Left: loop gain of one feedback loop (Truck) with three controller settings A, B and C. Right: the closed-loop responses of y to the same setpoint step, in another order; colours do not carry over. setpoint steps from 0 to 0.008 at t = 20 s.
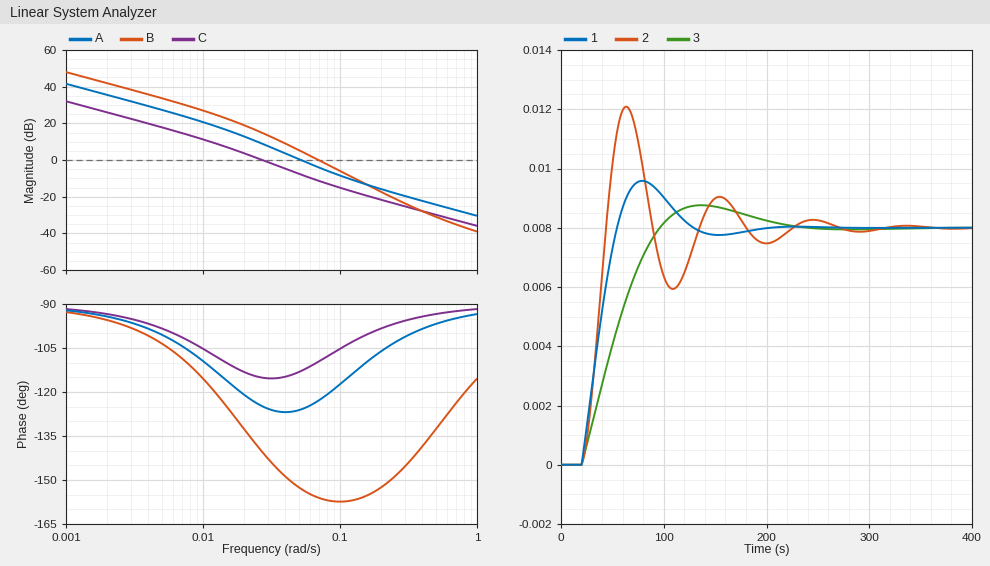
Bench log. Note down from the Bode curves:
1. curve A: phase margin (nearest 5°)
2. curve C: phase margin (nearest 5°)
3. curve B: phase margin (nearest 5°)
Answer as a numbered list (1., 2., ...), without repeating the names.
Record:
1. 55°
2. 65°
3. 25°
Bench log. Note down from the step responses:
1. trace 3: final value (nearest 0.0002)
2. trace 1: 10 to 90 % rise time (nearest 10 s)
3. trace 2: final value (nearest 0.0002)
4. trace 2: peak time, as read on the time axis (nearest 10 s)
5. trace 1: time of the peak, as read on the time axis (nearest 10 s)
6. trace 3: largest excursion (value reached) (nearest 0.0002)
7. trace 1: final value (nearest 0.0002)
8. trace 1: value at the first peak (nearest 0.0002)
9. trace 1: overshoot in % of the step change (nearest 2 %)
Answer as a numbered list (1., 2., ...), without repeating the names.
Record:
1. 0.0080
2. 30 s
3. 0.0080
4. 60 s
5. 80 s
6. 0.0088
7. 0.0080
8. 0.0096
9. 20 %
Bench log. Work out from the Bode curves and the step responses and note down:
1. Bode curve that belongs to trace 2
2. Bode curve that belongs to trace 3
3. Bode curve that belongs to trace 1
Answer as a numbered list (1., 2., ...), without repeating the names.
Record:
1. B
2. C
3. A
